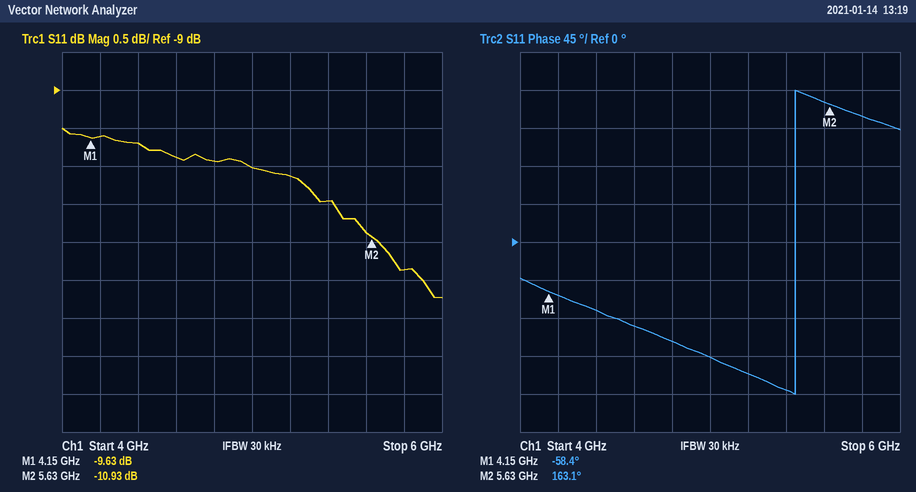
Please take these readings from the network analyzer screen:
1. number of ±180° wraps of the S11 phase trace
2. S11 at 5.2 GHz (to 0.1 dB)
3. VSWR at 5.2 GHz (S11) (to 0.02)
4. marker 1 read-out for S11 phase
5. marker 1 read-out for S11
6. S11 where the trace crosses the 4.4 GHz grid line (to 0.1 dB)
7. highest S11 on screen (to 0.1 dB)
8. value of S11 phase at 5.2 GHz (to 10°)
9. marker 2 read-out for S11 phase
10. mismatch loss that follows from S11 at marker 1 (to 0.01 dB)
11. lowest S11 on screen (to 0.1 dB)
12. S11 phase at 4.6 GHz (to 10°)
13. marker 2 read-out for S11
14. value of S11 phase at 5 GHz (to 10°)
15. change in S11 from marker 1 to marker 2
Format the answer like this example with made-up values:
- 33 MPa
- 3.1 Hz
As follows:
- 1
- -10.1 dB
- 1.90
- -58.4°
- -9.63 dB
- -9.7 dB
- -9.5 dB
- -160°
- 163.1°
- 0.50 dB
- -11.7 dB
- -100°
- -10.93 dB
- -140°
- -1.30 dB
